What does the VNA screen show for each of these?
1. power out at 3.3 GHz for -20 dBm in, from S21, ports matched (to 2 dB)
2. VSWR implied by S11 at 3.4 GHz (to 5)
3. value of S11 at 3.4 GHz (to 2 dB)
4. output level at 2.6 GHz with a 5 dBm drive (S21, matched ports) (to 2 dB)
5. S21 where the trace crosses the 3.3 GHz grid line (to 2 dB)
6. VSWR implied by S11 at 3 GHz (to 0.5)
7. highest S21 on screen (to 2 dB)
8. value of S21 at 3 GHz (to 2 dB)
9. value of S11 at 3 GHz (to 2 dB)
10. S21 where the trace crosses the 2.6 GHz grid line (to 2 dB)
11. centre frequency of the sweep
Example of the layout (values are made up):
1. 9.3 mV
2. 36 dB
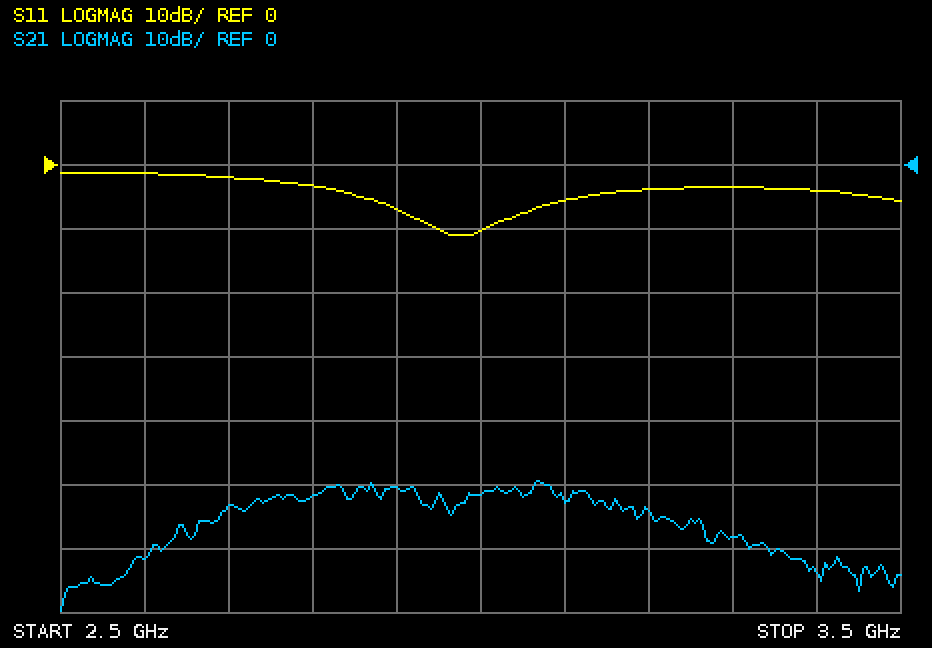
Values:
1. -78 dBm
2. 5
3. -4 dB
4. -56 dBm
5. -58 dB
6. 2.0
7. -50 dB
8. -52 dB
9. -10 dB
10. -62 dB
11. 3 GHz
